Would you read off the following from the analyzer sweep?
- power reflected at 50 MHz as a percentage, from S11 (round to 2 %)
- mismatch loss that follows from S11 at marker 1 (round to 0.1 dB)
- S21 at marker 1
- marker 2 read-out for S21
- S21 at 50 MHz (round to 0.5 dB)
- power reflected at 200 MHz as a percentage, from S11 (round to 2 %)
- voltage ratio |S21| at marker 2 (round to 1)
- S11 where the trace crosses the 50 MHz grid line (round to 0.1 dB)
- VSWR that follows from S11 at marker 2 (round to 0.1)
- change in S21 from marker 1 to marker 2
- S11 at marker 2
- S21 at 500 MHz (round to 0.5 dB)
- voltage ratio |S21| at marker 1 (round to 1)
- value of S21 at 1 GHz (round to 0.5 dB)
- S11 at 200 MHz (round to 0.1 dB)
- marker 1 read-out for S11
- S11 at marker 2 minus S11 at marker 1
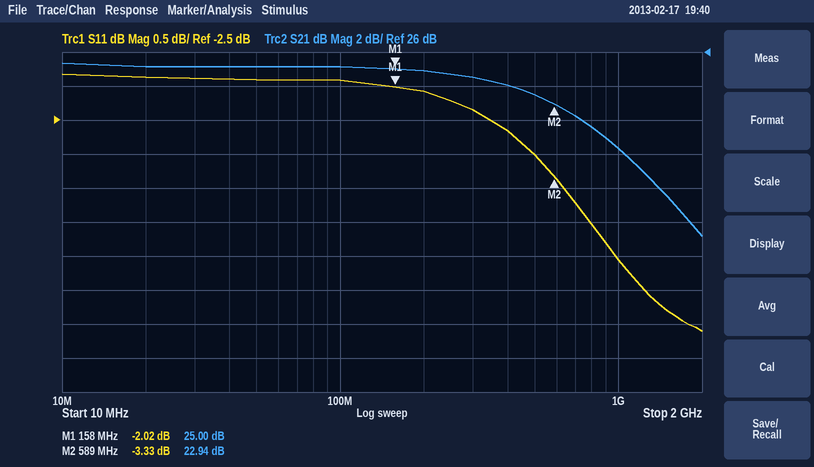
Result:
64 %
4.3 dB
25.00 dB
22.94 dB
25.0 dB
62 %
14
-1.9 dB
5.3
-2.06 dB
-3.33 dB
23.5 dB
18
20.5 dB
-2.1 dB
-2.02 dB
-1.31 dB
